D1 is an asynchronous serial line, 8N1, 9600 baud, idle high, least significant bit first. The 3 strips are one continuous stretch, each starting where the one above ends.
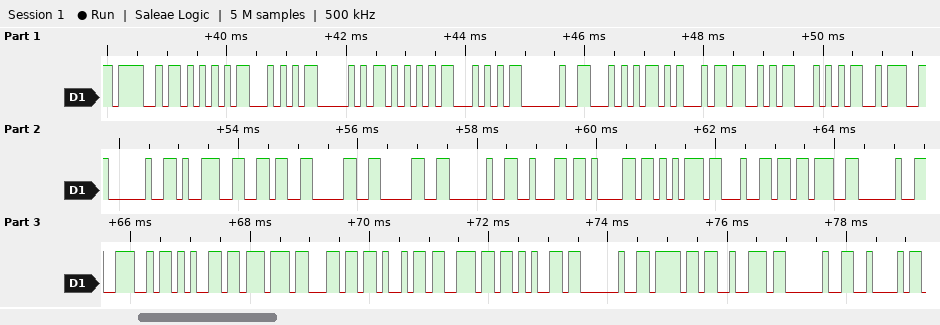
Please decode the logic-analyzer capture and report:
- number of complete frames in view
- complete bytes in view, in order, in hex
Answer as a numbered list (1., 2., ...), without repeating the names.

1. 36
2. 4F 55 54 50 55 54 20 54 45 53 54 3A 20 39 36 30 30 20 62 61 75 64 3B 20 4E 65 77 6C 69 6E 65 20 6F 72 20 42
